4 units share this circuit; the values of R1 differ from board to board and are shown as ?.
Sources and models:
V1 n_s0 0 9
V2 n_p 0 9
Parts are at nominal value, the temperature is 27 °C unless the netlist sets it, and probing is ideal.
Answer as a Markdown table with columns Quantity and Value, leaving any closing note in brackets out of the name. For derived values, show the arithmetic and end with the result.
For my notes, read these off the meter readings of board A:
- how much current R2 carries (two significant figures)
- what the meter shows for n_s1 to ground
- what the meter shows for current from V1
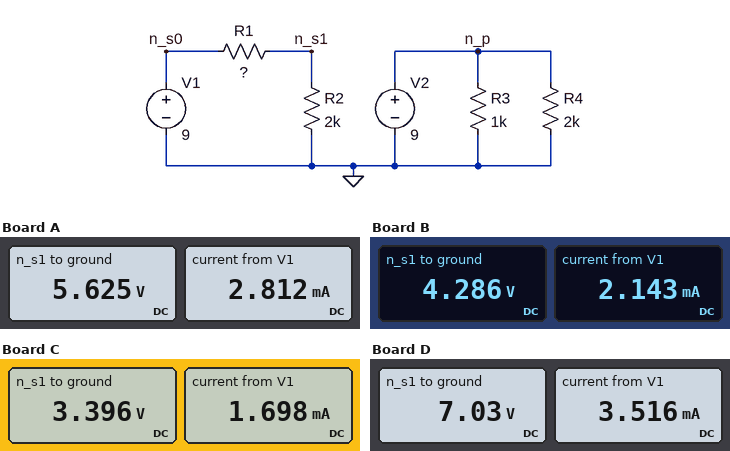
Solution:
| Quantity | Value |
|---|---|
| how much current R2 carries | (5.625 V) / 2 kΩ = 2.8 mA |
| what the meter shows for n_s1 to ground | 5.625 V |
| what the meter shows for current from V1 | 2.812 mA |
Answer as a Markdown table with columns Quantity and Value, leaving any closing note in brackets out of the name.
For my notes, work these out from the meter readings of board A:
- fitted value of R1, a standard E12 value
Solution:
| Quantity | Value |
|---|---|
| fitted value of R1, a standard E12 value | 1.2 kΩ |
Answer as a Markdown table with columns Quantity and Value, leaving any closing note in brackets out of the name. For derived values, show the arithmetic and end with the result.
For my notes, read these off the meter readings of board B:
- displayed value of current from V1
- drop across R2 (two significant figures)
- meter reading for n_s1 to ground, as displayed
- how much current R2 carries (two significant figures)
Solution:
| Quantity | Value |
|---|---|
| displayed value of current from V1 | 2.143 mA |
| drop across R2 | 4.286 V = 4.3 V |
| meter reading for n_s1 to ground, as displayed | 4.286 V |
| how much current R2 carries | (4.286 V) / 2 kΩ = 2.1 mA |
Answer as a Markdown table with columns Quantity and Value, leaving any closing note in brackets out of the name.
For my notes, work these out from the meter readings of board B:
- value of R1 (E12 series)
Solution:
| Quantity | Value |
|---|---|
| value of R1 | 2.2 kΩ |
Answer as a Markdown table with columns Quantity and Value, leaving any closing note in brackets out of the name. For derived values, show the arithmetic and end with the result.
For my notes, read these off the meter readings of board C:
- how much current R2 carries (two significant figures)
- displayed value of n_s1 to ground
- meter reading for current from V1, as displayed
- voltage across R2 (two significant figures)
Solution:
| Quantity | Value |
|---|---|
| how much current R2 carries | (3.396 V) / 2 kΩ = 1.7 mA |
| displayed value of n_s1 to ground | 3.396 V |
| meter reading for current from V1, as displayed | 1.698 mA |
| voltage across R2 | 3.396 V = 3.4 V |
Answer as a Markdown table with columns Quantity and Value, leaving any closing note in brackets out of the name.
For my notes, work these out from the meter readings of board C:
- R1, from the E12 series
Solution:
| Quantity | Value |
|---|---|
| R1, from the E12 series | 3.3 kΩ |
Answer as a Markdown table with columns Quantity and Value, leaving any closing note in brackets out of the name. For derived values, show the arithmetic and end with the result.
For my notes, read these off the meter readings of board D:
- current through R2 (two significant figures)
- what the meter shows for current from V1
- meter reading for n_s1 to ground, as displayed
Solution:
| Quantity | Value |
|---|---|
| current through R2 | (7.03 V) / 2 kΩ = 3.5 mA |
| what the meter shows for current from V1 | 3.516 mA |
| meter reading for n_s1 to ground, as displayed | 7.03 V |
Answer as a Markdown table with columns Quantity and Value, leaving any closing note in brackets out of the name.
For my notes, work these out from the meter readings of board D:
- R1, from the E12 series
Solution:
| Quantity | Value |
|---|---|
| R1, from the E12 series | 560 Ω |
